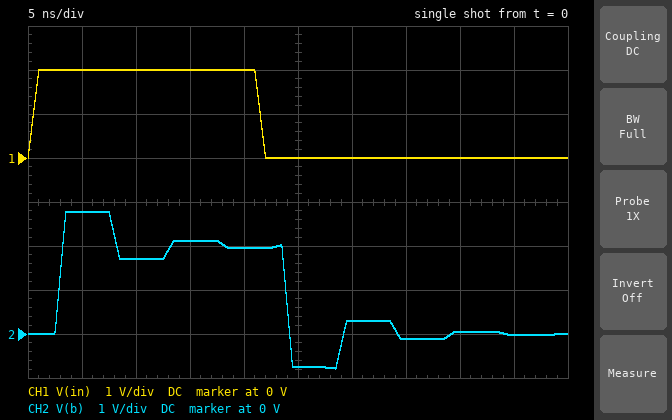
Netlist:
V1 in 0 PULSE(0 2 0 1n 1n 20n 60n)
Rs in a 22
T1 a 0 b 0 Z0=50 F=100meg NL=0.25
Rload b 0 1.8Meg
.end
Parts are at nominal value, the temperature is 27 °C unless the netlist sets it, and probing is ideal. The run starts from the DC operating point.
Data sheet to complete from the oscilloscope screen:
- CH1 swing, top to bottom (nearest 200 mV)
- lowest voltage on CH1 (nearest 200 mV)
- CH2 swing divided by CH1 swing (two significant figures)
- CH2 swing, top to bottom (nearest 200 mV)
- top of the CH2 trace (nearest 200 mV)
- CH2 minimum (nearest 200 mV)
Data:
2.0 V
0 V
1.8
3.6 V
2.8 V
-800 mV
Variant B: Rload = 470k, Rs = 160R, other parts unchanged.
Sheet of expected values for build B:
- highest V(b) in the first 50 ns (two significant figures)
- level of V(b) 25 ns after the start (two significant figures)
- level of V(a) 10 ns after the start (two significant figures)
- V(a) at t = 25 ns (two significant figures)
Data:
1.9 V
970 mV
1.2 V
1.4 V
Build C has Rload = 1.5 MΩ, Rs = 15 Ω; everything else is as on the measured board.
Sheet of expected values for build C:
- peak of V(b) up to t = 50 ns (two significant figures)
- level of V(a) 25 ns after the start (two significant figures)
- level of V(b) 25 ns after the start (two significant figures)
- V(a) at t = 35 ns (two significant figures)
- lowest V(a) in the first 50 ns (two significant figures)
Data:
3.1 V
420 mV
-990 mV
120 mV
-260 mV
